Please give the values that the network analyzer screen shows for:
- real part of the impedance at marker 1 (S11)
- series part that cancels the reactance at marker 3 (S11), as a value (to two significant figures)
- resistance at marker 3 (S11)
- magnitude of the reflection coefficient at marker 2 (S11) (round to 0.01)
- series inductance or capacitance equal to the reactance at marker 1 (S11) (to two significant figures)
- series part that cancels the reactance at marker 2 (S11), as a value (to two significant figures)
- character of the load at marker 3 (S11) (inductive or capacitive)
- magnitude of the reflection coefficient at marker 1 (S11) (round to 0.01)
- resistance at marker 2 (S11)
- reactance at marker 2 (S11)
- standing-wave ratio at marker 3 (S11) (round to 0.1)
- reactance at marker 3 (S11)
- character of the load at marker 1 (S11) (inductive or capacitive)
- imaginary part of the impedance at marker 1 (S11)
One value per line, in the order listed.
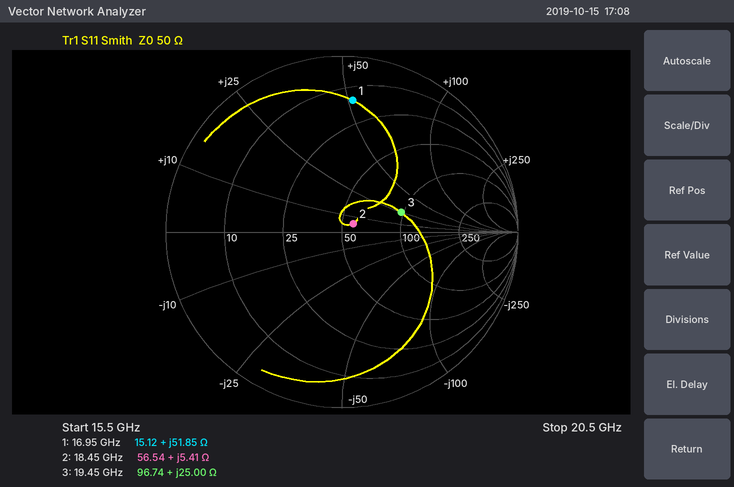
15.12 Ω
330 fF
96.74 Ω
0.08
490 pH
1.6 pF
inductive
0.75
56.54 Ω
+5.41 Ω
2.1
+25.00 Ω
inductive
+51.85 Ω
